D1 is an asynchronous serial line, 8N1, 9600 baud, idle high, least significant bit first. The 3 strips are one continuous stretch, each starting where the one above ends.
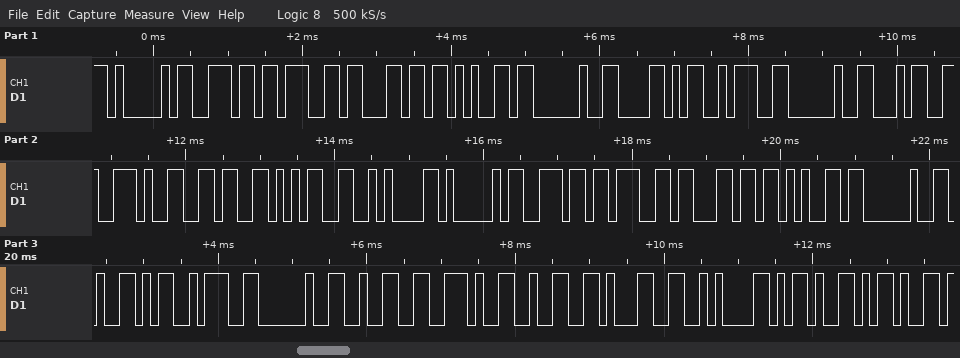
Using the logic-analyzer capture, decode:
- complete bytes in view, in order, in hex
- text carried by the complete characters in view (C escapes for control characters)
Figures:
41 6E 67 6C 65 20 58 3A 20 34 2E 36 35 0A 41 6E 67 6C 65 20 59 3A 20 32 2E 32 31 0A 2D 2D
"Angle X: 4.65\nAngle Y: 2.21\n--"
